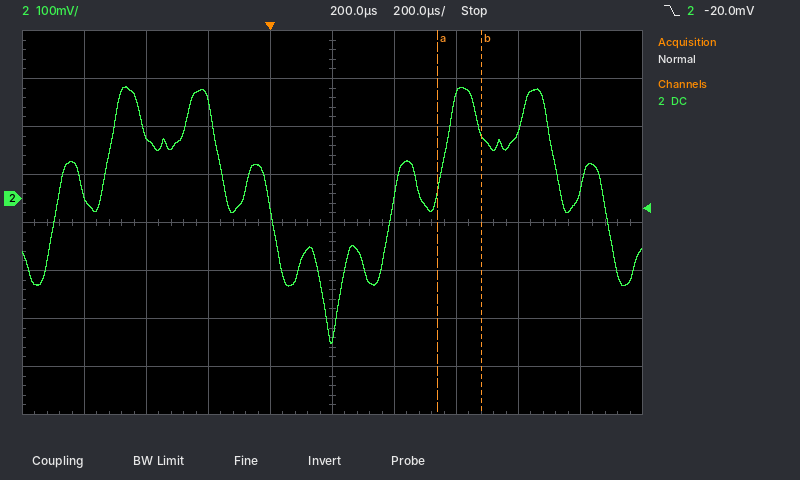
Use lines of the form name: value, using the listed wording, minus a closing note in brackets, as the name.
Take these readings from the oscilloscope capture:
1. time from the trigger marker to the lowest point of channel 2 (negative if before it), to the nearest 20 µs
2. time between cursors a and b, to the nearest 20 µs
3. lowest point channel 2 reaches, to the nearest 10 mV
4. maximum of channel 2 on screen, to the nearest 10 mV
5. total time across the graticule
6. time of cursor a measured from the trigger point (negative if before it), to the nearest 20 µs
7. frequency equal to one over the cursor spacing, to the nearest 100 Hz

time from the trigger marker to the lowest point of channel 2 (negative if before it), to the nearest 20 µs: +200 µs
time between cursors a and b, to the nearest 20 µs: 140 µs
lowest point channel 2 reaches, to the nearest 10 mV: -300 mV
maximum of channel 2 on screen, to the nearest 10 mV: 230 mV
total time across the graticule: 2 ms
time of cursor a measured from the trigger point (negative if before it), to the nearest 20 µs: +540 µs
frequency equal to one over the cursor spacing, to the nearest 100 Hz: 7.1 kHz
